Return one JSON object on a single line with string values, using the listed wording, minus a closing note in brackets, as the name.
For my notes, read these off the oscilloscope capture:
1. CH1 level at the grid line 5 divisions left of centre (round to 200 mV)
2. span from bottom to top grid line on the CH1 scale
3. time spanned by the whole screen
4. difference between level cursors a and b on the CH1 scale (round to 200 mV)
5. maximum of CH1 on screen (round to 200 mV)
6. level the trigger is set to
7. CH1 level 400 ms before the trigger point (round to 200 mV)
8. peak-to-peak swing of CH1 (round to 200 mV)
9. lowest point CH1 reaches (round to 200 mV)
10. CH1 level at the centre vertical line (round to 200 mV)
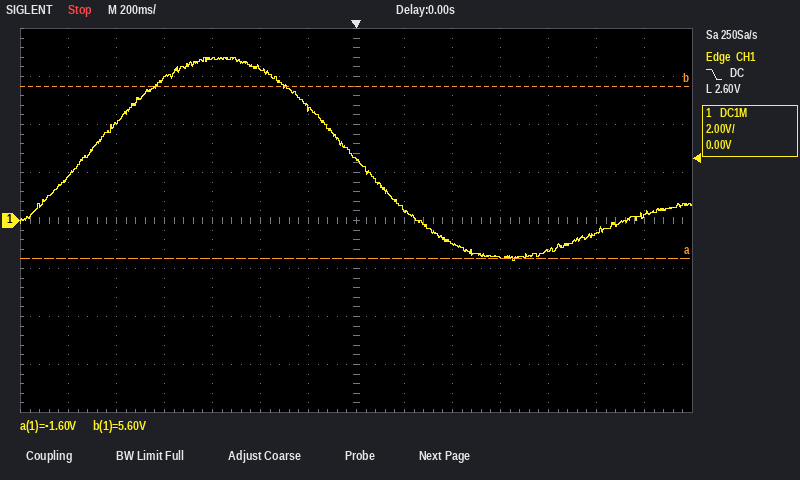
{"CH1 level at the grid line 5 divisions left of centre": "4.0 V", "span from bottom to top grid line on the CH1 scale": "16 V", "time spanned by the whole screen": "2.8 s", "difference between level cursors a and b on the CH1 scale": "7.2 V", "maximum of CH1 on screen": "6.8 V", "level the trigger is set to": "2.60 V", "CH1 level 400 ms before the trigger point": "6.4 V", "peak-to-peak swing of CH1": "8.4 V", "lowest point CH1 reaches": "-1.6 V", "CH1 level at the centre vertical line": "2.6 V"}
